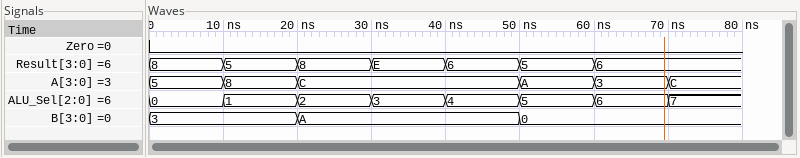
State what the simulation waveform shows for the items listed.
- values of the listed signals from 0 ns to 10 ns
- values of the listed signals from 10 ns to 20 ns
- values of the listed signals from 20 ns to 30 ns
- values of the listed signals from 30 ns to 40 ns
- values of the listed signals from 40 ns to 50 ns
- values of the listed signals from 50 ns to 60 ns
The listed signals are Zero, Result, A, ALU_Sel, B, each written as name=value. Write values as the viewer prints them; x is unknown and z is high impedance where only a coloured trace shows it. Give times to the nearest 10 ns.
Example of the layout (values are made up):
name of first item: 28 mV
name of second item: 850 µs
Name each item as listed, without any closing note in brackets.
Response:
values of the listed signals from 0 ns to 10 ns: Zero=0, Result=8, A=5, ALU_Sel=0, B=3
values of the listed signals from 10 ns to 20 ns: Zero=0, Result=5, A=8, ALU_Sel=1, B=3
values of the listed signals from 20 ns to 30 ns: Zero=0, Result=8, A=C, ALU_Sel=2, B=A
values of the listed signals from 30 ns to 40 ns: Zero=0, Result=E, A=C, ALU_Sel=3, B=A
values of the listed signals from 40 ns to 50 ns: Zero=0, Result=6, A=C, ALU_Sel=4, B=A
values of the listed signals from 50 ns to 60 ns: Zero=0, Result=5, A=A, ALU_Sel=5, B=0
